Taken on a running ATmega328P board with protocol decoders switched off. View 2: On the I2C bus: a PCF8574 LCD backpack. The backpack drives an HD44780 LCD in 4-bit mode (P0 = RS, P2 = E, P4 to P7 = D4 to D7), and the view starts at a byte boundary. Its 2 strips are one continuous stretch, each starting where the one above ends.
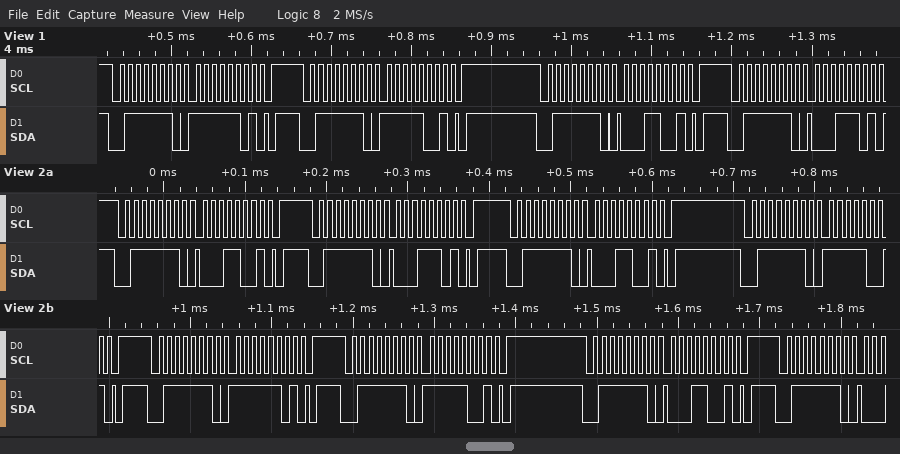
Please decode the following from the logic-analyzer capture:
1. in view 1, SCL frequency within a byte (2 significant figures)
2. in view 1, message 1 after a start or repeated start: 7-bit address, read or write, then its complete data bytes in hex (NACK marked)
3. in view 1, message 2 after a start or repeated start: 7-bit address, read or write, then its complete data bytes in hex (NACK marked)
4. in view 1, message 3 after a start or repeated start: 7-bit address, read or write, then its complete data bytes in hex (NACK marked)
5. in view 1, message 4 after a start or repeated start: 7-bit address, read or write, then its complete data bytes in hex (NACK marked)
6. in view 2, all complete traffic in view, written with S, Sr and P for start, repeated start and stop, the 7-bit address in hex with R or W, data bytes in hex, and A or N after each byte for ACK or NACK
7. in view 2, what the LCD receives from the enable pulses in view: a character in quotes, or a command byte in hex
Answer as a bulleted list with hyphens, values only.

- 100 kHz
- 0x3F write: FD
- 0x3F write: F9
- 0x3F write: 19
- 0x3F write: 1D
- S 3FW A 19 A P S 3FW A 1D A P S 3FW A 19 A P S 3FW A F9 A P S 3FW A FD A P S 3FW A F9 A P S 3FW A 19 A P S 3FW A
- data 0x1F
